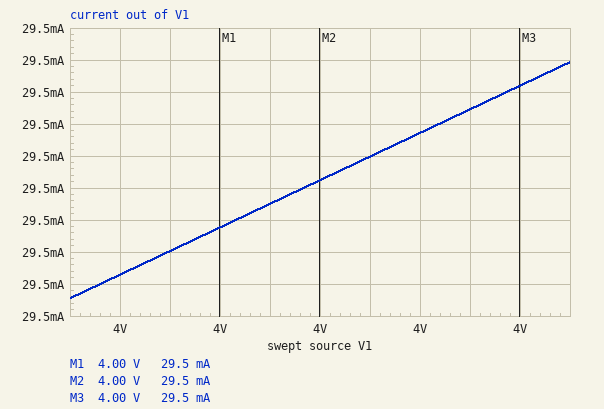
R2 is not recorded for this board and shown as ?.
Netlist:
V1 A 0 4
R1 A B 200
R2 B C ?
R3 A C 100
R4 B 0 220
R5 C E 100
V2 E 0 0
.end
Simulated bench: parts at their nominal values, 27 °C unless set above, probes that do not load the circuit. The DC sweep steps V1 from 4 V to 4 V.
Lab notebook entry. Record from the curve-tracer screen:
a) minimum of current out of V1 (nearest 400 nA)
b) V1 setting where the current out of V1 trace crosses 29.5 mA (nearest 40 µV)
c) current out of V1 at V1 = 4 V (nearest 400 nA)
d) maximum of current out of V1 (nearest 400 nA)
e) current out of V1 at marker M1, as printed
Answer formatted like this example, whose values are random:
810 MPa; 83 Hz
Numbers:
29.5212 mA; 3.99940 V; 29.5344 mA; 29.5360 mA; 29.5 mA
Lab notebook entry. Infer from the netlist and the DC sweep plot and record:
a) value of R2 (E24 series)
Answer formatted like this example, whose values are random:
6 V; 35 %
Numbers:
330 Ω
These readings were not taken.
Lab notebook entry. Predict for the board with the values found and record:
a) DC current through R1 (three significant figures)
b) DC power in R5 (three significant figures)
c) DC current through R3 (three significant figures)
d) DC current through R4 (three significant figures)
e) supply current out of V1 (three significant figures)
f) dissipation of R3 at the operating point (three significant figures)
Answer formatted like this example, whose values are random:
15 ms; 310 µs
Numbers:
9.63 mA; 40.4 mW; 19.9 mA; 9.43 mA; 29.5 mA; 39.6 mW
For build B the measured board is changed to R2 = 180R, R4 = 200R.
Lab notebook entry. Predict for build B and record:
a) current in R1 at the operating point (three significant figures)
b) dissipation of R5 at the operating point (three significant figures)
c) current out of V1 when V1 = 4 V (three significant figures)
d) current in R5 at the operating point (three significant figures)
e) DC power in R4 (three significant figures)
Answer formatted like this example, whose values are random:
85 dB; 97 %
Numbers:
10.0 mA; 40.0 mW; 30.0 mA; 20.0 mA; 20.0 mW
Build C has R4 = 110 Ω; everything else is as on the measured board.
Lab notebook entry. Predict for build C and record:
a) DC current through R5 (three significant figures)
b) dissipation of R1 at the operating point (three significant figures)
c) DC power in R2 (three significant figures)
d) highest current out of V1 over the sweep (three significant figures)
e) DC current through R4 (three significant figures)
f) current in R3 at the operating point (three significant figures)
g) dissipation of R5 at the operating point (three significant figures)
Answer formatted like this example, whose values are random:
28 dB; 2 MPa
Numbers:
19.4 mA; 31.0 mW; 547 µW; 33.1 mA; 13.7 mA; 20.6 mA; 37.5 mW
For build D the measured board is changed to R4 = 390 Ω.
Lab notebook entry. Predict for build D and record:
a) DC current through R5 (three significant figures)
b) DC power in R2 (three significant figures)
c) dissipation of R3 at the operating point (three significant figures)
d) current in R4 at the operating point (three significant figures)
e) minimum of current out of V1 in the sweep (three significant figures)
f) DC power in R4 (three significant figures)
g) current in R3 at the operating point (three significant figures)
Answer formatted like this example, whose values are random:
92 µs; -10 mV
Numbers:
20.6 mA; 522 µW; 37.5 mW; 6.35 mA; 27.0 mA; 15.7 mW; 19.4 mA
